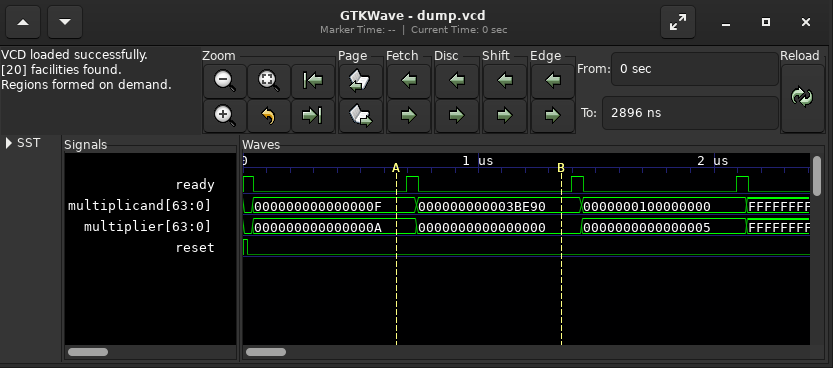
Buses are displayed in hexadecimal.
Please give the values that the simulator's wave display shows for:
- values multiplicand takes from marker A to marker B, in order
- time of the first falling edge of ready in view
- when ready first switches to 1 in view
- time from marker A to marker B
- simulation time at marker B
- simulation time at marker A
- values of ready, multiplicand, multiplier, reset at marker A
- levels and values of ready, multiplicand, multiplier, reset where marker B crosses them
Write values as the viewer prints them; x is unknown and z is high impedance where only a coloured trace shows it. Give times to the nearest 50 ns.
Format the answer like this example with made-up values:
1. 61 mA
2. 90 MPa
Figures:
1. 000000000000000F, 000000000003BE90
2. 50 ns
3. 700 ns
4. 700 ns
5. 1350 ns
6. 650 ns
7. ready=0, multiplicand=000000000000000F, multiplier=000000000000000A, reset=0
8. ready=0, multiplicand=000000000003BE90, multiplier=0000000000000000, reset=0
